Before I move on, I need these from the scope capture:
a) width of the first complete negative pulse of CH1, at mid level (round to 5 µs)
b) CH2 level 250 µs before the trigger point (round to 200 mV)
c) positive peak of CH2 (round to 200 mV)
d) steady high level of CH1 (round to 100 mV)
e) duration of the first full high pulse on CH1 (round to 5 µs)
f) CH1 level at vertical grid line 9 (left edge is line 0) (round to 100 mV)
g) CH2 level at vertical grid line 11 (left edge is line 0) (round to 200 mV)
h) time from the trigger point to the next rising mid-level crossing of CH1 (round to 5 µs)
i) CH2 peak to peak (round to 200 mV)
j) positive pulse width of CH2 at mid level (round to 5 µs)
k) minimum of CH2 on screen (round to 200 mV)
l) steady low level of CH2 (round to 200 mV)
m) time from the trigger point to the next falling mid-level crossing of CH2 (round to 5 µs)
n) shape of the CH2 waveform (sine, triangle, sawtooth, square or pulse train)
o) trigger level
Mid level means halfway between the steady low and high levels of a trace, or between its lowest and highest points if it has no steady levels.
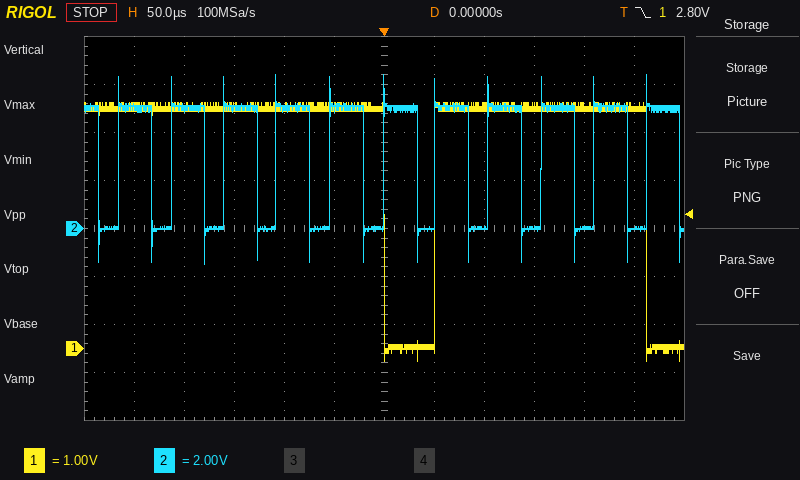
50 µs
5.0 V
6.4 V
5.0 V
210 µs
5.0 V
0.0 V
50 µs
7.8 V
35 µs
-1.4 V
0.0 V
35 µs
pulse train
2.80 V
